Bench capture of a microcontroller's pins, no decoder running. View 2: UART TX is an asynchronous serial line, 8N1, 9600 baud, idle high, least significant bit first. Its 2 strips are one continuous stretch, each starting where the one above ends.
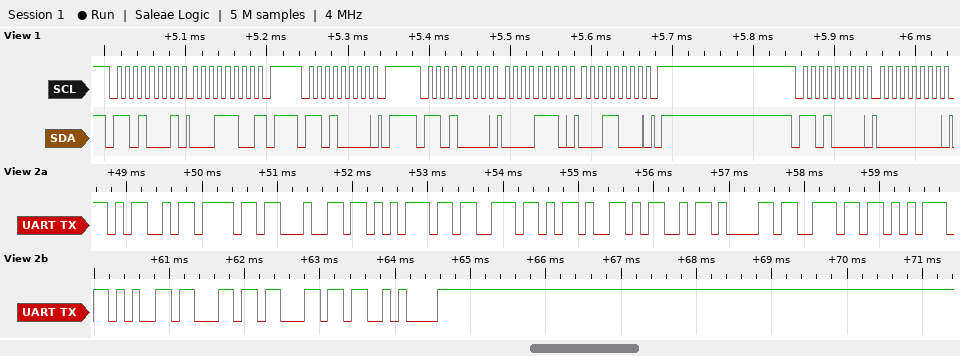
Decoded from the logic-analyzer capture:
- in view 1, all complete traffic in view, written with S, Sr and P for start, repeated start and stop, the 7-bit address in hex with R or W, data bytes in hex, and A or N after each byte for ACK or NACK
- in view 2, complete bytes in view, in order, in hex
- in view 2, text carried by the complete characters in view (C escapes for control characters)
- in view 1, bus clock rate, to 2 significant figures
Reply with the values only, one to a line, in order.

S 68R A 1C N P S 68W A P S 68W A 0E A 18 A P S 68W A 00 A
0x4D 0x6F 0x64 0x75 0x73 0x2D 0x4D 0x61 0x6E 0x75 0x65 0x6C 0x6C 0x0A
"Modus-Manuell\n"
100 kHz
